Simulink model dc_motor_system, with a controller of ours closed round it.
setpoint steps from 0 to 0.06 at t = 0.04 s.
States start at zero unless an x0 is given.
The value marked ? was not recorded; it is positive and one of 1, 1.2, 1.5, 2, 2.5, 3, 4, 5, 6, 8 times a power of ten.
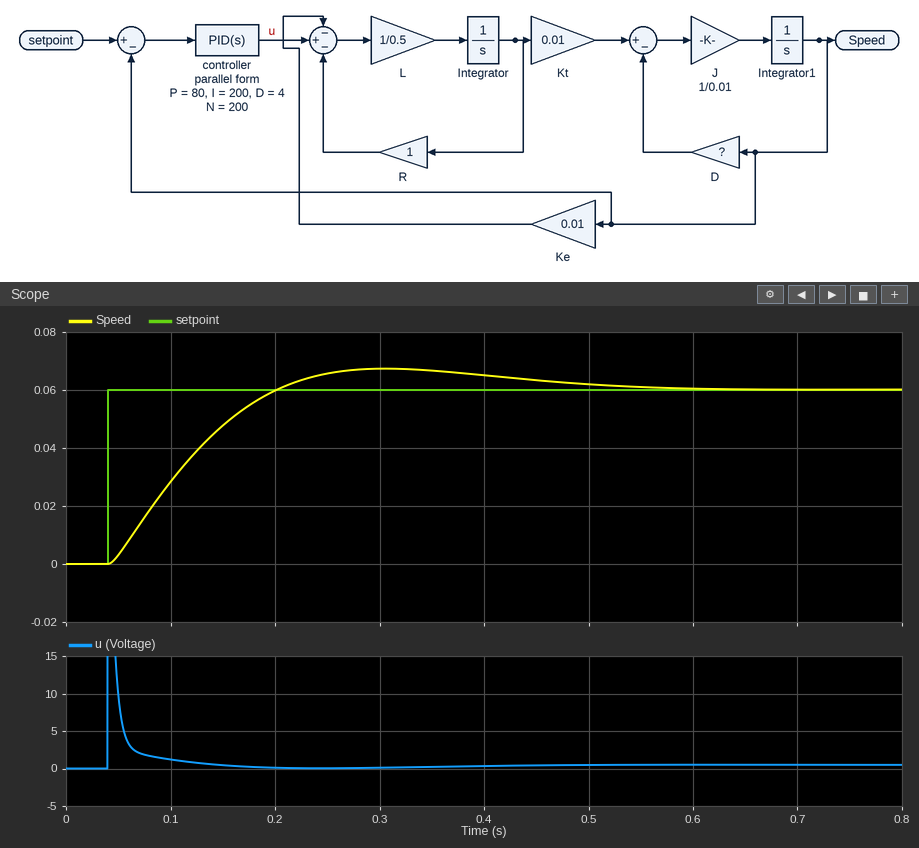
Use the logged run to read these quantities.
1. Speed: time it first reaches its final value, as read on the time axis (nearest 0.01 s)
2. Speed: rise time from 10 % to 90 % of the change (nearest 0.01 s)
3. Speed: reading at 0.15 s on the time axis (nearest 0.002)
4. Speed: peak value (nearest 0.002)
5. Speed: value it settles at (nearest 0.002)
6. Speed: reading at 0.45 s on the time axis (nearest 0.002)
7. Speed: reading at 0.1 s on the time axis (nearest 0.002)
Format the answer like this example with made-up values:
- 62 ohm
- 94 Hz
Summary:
- 0.20 s
- 0.12 s
- 0.048
- 0.068
- 0.060
- 0.064
- 0.028
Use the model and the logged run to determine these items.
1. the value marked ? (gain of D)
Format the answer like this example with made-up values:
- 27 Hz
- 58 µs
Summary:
- 0.08
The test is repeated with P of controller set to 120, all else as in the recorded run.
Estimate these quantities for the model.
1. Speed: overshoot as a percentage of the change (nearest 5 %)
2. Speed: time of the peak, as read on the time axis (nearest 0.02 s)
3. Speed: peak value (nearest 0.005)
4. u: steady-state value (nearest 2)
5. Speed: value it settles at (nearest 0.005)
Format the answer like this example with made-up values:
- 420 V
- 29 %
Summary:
- 15 %
- 0.24 s
- 0.070
- 0
- 0.060
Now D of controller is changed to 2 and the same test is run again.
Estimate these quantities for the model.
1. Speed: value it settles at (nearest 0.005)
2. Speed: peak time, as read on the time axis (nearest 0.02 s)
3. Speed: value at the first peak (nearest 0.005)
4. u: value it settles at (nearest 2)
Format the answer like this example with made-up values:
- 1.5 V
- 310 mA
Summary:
- 0.060
- 0.30 s
- 0.075
- 0
